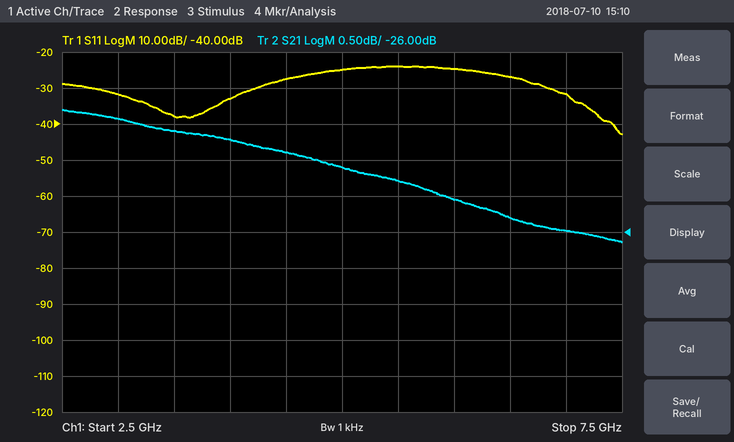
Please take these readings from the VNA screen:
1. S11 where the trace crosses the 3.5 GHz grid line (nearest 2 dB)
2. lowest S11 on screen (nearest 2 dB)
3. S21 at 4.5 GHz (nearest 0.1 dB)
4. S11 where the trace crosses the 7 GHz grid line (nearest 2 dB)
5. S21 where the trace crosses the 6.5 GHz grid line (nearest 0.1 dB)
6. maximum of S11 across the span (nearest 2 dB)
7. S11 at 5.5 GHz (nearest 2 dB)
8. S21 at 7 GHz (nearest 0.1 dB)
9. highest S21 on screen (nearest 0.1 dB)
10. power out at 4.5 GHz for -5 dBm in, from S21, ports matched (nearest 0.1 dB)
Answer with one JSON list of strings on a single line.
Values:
["-38 dB", "-42 dB", "-24.9 dB", "-32 dB", "-25.8 dB", "-24 dB", "-24 dB", "-26.0 dB", "-24.3 dB", "-29.9 dBm"]
